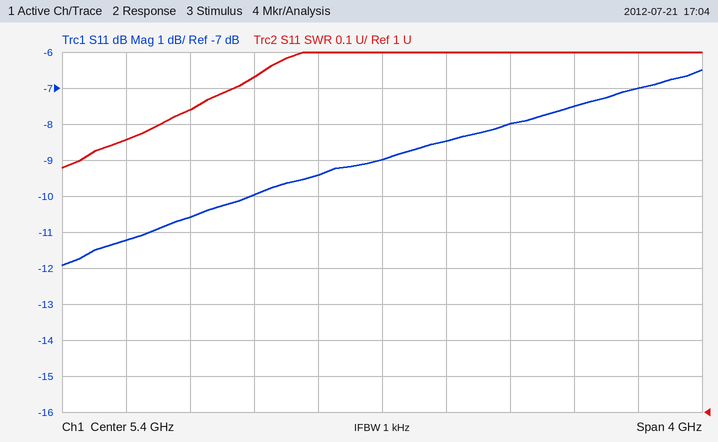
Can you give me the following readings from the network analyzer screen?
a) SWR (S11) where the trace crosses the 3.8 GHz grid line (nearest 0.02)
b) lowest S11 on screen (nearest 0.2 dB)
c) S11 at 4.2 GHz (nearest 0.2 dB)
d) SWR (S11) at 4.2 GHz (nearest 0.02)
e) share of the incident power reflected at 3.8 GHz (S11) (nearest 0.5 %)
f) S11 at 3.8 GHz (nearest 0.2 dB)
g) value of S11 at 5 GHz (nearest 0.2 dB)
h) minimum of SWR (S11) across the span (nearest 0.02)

1.76
-12.0 dB
-10.6 dB
1.84
7.5 %
-11.2 dB
-9.4 dB
1.68
